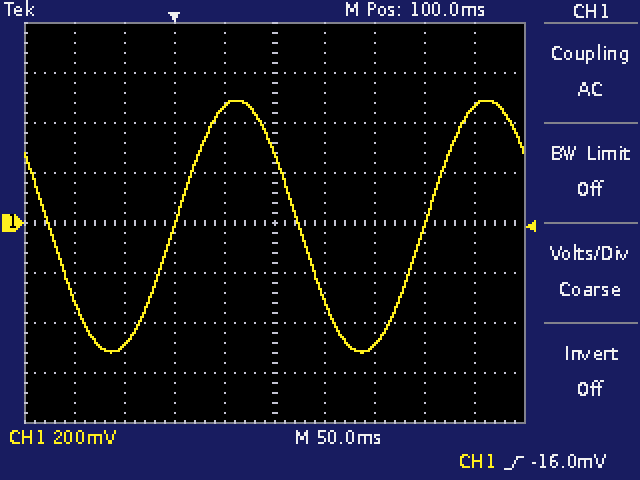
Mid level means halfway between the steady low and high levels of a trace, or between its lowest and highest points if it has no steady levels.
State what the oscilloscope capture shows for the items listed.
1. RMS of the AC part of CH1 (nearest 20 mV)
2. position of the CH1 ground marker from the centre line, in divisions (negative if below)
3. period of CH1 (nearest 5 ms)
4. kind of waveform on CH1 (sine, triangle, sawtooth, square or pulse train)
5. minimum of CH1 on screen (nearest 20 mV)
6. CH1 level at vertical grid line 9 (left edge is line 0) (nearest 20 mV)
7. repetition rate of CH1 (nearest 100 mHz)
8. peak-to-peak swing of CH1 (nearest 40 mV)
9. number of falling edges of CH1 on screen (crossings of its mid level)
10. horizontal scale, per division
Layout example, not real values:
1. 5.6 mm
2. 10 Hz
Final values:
1. 360 mV
2. 0.0 div
3. 250 ms
4. sine
5. -520 mV
6. 460 mV
7. 4.0 Hz
8. 1.00 V
9. 2
10. 50 ms
